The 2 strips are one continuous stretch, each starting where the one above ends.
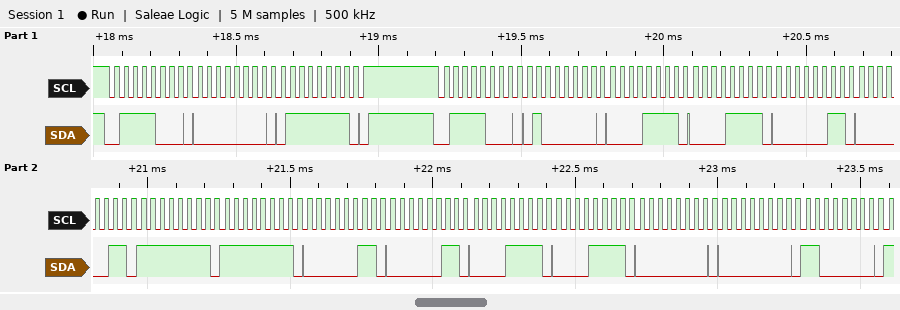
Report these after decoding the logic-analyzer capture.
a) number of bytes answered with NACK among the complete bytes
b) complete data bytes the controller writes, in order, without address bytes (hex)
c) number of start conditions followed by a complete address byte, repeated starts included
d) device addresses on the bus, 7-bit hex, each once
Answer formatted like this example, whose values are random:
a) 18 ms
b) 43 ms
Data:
a) 0
b) 00 7F 40 0F 0F 03 03 FF FF 03 03 0F 0F 00 00 C0
c) 2
d) 0x3C
